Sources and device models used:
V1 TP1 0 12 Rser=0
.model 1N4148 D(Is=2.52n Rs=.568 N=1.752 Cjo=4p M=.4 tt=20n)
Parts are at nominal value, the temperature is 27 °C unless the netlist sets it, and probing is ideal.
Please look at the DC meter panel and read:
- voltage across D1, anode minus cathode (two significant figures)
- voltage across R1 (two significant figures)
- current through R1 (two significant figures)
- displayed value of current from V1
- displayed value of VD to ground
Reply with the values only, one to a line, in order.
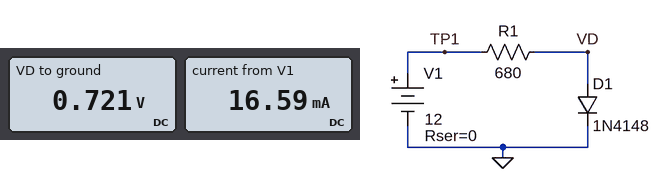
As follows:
720 mV
11 V
17 mA
16.59 mA
0.721 V
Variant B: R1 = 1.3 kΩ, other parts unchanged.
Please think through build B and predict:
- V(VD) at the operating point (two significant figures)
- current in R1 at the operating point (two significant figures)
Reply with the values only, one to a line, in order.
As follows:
690 mV
8.7 mA
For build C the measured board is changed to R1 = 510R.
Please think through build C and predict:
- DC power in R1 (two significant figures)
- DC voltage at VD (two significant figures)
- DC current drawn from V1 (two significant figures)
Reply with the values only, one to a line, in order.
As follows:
250 mW
740 mV
22 mA
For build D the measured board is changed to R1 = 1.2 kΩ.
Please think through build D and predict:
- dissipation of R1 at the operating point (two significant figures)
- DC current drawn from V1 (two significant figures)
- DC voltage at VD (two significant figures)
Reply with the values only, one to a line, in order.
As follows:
110 mW
9.4 mA
690 mV
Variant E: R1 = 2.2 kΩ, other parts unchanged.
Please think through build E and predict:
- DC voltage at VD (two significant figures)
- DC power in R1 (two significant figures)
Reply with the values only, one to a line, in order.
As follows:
660 mV
58 mW
